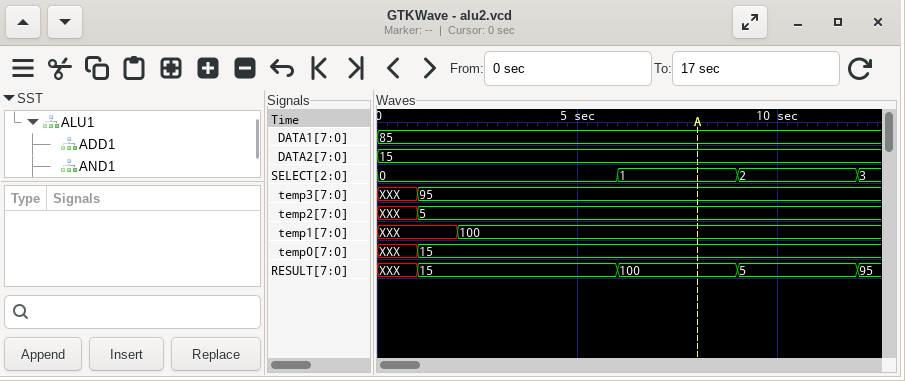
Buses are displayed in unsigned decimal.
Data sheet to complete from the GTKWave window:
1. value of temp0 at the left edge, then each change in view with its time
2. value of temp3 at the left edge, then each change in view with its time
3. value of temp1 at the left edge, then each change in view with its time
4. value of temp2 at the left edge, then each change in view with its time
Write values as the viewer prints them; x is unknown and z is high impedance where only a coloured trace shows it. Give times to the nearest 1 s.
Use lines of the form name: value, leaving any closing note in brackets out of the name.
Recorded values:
value of temp0 at the left edge, then each change in view with its time: XXX, 15 at 1 s
value of temp3 at the left edge, then each change in view with its time: XXX, 95 at 1 s
value of temp1 at the left edge, then each change in view with its time: XXX, 100 at 2 s
value of temp2 at the left edge, then each change in view with its time: XXX, 5 at 1 s
